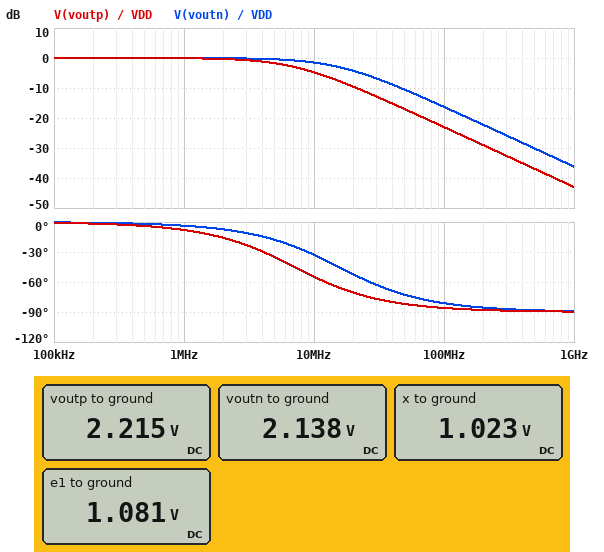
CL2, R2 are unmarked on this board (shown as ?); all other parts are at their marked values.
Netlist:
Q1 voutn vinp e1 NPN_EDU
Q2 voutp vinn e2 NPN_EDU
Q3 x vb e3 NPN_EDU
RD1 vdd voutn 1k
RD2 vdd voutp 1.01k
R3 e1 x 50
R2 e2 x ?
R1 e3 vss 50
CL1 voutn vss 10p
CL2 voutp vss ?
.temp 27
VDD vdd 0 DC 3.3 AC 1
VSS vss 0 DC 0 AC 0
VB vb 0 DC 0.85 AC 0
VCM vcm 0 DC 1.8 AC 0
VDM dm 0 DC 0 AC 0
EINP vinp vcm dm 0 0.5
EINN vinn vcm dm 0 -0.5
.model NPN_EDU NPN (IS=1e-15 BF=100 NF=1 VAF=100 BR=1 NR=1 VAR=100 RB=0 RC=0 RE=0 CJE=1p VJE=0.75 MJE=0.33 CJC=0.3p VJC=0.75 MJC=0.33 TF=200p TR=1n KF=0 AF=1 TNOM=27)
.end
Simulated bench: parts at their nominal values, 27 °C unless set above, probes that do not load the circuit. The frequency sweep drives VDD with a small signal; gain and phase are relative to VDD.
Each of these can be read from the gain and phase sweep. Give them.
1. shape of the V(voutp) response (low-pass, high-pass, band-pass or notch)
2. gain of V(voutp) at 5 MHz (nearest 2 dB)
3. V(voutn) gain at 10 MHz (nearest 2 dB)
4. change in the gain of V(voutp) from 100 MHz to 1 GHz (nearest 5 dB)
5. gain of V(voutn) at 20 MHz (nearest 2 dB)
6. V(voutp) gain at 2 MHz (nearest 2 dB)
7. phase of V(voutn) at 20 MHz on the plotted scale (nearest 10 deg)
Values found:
low-pass
-2 dB
-2 dB
-20 dB
-4 dB
0 dB
-50 deg
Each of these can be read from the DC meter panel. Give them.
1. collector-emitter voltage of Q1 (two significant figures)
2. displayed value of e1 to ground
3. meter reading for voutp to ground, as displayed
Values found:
1.1 V
1.081 V
2.215 V
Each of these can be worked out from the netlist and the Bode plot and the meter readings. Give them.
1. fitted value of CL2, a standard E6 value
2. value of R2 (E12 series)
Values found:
22 pF
56 Ω
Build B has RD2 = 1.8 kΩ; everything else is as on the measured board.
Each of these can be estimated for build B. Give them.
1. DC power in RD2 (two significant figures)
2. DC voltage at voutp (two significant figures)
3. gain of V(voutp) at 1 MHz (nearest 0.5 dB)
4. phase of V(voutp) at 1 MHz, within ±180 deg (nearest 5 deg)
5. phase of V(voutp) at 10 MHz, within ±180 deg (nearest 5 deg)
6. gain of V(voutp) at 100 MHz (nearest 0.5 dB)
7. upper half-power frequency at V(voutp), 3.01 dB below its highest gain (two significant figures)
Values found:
2.1 mW
1.4 V
-0.5 dB
-15 deg
-70 deg
-28.0 dB
4.0 MHz
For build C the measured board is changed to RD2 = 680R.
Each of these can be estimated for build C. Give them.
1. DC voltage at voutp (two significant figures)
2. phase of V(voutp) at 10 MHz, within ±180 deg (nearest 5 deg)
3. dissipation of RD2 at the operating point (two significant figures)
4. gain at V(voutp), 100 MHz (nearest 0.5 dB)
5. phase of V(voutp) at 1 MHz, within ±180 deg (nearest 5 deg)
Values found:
2.6 V
-45 deg
790 µW
-19.5 dB
-5 deg
